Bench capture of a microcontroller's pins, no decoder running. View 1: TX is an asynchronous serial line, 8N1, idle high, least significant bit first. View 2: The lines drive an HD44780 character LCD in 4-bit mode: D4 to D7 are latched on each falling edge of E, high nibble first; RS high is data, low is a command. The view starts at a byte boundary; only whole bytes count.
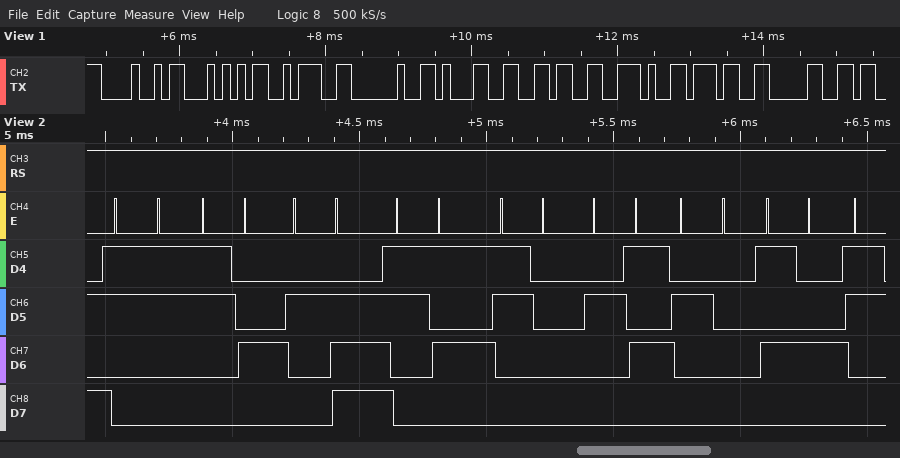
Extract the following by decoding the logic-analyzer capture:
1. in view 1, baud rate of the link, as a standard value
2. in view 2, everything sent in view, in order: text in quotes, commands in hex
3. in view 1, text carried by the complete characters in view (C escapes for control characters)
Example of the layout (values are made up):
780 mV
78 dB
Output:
9600 baud
"34.50% T"
"HT: 16.70"
